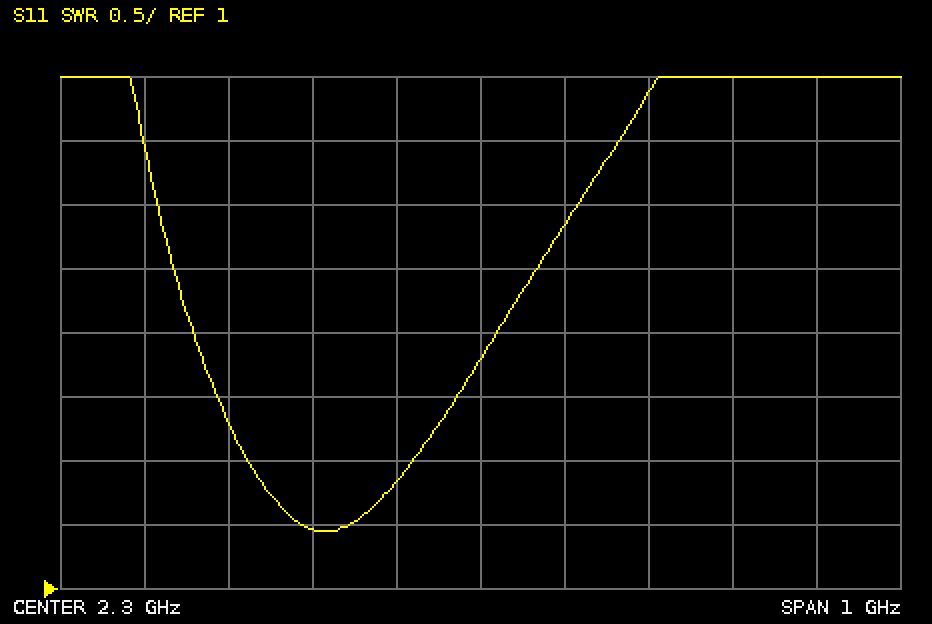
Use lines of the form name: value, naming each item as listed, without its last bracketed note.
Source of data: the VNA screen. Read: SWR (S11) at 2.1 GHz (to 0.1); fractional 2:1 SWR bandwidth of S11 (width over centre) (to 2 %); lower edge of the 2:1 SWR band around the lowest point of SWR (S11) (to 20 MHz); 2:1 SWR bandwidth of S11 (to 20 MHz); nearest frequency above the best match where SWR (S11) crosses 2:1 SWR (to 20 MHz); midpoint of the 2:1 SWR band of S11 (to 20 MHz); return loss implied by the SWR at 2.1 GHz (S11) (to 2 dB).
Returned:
SWR (S11) at 2.1 GHz: 1.5
fractional 2:1 SWR bandwidth of S11 (width over centre): 10 %
lower edge of the 2:1 SWR band around the lowest point of SWR (S11): 2.02 GHz
2:1 SWR bandwidth of S11: 200 MHz
nearest frequency above the best match where SWR (S11) crosses 2:1 SWR: 2.22 GHz
midpoint of the 2:1 SWR band of S11: 2.12 GHz
return loss implied by the SWR at 2.1 GHz (S11): 14 dB
